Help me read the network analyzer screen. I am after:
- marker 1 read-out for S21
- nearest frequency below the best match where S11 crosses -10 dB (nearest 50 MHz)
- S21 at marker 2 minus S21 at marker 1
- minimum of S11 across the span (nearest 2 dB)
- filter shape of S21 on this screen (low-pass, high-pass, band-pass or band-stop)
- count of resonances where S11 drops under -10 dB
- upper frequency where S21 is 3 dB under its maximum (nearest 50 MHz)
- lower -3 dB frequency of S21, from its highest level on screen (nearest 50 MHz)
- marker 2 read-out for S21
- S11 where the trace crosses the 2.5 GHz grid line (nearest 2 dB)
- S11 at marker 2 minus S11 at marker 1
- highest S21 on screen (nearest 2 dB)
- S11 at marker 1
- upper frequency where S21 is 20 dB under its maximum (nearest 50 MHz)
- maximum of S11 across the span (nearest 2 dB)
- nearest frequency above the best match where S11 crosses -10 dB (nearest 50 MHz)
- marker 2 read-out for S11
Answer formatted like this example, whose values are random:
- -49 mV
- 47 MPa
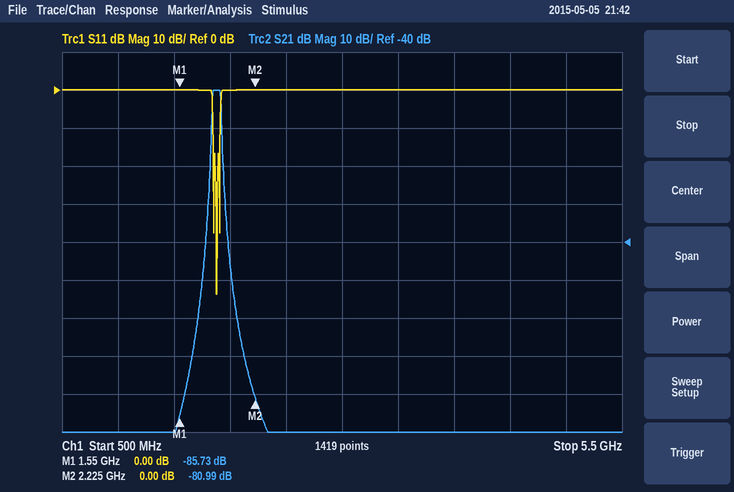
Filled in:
- -85.73 dB
- 1.85 GHz
- 4.74 dB
- -54 dB
- band-pass
- 3
- 1.90 GHz
- 1.85 GHz
- -80.99 dB
- 0 dB
- 0.00 dB
- 0 dB
- 0.00 dB
- 1.95 GHz
- 0 dB
- 1.90 GHz
- 0.00 dB
